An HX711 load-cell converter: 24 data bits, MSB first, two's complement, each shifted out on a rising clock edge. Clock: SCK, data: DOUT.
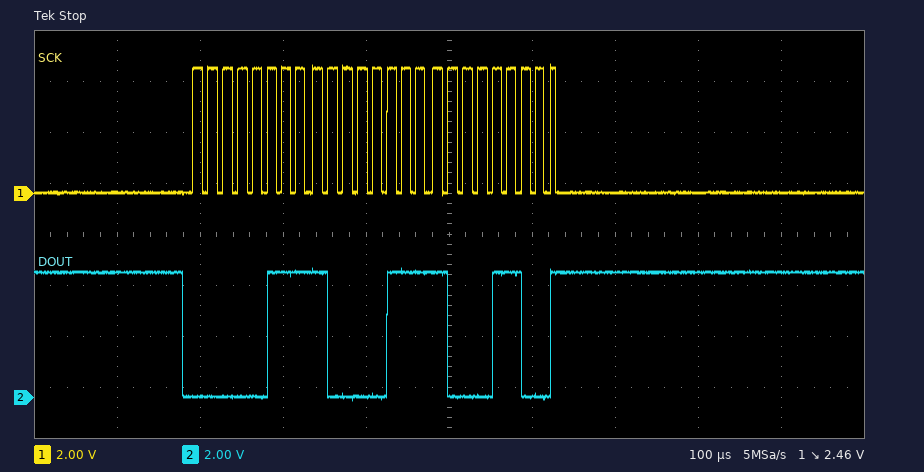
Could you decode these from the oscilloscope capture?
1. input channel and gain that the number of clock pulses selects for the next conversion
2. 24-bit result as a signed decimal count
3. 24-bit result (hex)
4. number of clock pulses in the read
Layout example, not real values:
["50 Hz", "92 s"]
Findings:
["channel A, gain 128", "493452", "0x07878C", "25"]
